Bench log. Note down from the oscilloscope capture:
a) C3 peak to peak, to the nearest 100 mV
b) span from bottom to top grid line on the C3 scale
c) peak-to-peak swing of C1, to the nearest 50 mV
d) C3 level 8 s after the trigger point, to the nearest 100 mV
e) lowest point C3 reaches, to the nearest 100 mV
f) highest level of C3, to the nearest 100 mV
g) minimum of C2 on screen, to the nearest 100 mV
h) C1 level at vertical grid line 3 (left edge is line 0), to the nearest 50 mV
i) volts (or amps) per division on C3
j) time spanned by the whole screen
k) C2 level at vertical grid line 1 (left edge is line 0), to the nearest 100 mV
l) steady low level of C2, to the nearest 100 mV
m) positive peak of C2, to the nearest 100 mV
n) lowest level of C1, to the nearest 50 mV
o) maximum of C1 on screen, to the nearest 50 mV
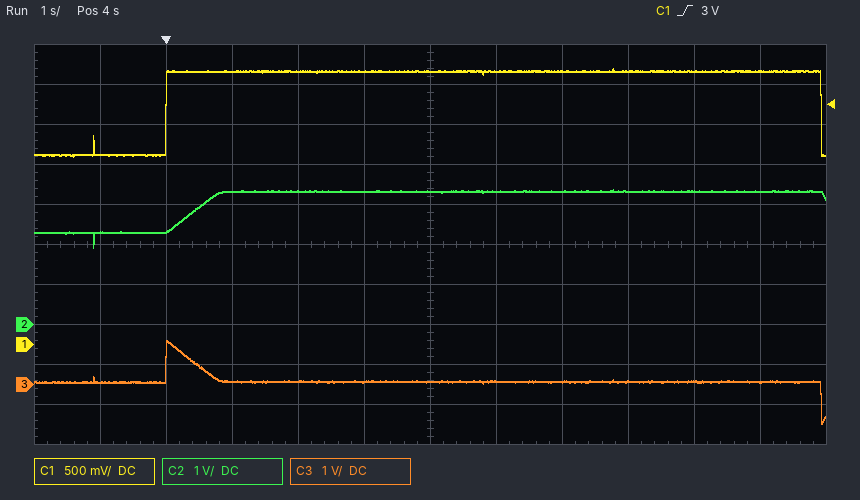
2.1 V
10 V
1.10 V
100 mV
-1.0 V
1.1 V
1.9 V
3.40 V
1 V
12 s
2.3 V
2.3 V
3.4 V
2.35 V
3.45 V
